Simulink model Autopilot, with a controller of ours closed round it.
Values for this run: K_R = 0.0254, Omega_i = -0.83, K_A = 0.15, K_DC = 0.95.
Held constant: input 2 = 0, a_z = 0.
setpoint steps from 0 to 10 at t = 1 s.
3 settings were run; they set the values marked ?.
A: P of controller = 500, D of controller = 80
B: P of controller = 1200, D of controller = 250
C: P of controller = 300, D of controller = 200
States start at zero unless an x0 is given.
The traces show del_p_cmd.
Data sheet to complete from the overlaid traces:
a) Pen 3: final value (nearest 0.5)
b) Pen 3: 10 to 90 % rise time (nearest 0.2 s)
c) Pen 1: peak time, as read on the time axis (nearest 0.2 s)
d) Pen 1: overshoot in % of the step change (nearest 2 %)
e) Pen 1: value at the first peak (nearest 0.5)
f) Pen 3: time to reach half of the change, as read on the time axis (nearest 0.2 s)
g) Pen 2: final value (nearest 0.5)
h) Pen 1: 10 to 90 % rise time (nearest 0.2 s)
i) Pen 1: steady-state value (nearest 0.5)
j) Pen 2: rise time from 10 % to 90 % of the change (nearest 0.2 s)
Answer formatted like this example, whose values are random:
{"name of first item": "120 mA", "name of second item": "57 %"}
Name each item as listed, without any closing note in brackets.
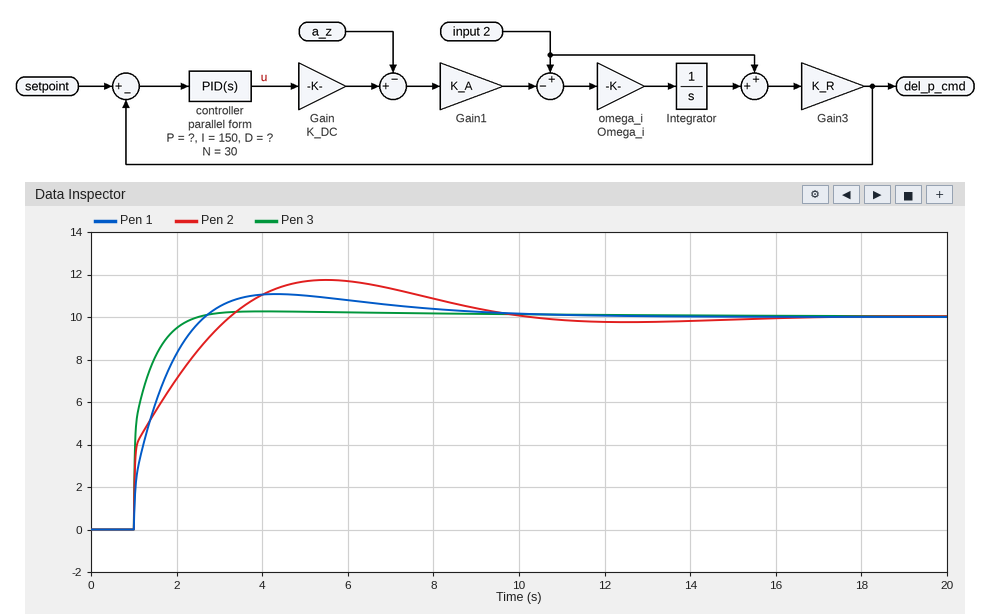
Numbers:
{"Pen 3: final value": "10.0", "Pen 3: 10 to 90 % rise time": "0.8 s", "Pen 1: peak time, as read on the time axis": "4.4 s", "Pen 1: overshoot in % of the step change": "10 %", "Pen 1: value at the first peak": "11.0", "Pen 3: time to reach half of the change, as read on the time axis": "1.0 s", "Pen 2: final value": "10.0", "Pen 1: 10 to 90 % rise time": "1.2 s", "Pen 1: steady-state value": "10.0", "Pen 2: rise time from 10 % to 90 % of the change": "1.8 s"}
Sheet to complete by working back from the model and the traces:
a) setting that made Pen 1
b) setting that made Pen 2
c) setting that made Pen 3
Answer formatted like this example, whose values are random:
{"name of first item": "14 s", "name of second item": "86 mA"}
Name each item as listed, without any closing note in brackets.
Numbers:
{"setting that made Pen 1": "A", "setting that made Pen 2": "C", "setting that made Pen 3": "B"}
